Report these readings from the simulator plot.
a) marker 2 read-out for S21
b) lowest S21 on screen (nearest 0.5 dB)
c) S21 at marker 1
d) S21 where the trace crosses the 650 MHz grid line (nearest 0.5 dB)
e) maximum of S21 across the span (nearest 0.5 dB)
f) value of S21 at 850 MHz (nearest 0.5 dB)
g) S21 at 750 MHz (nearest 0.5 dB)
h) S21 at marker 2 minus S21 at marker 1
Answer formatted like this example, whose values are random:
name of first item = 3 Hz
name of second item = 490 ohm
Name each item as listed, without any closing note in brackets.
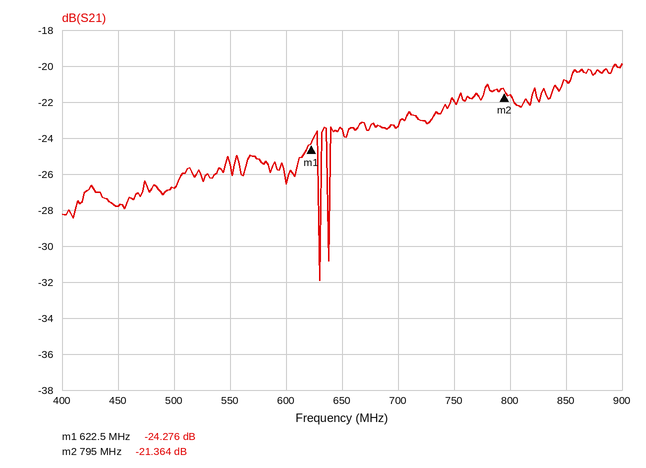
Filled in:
marker 2 read-out for S21 = -21.364 dB
lowest S21 on screen = -32.0 dB
S21 at marker 1 = -24.276 dB
S21 where the trace crosses the 650 MHz grid line = -23.5 dB
maximum of S21 across the span = -20.0 dB
value of S21 at 850 MHz = -21.0 dB
S21 at 750 MHz = -22.0 dB
S21 at marker 2 minus S21 at marker 1 = 2.912 dB
